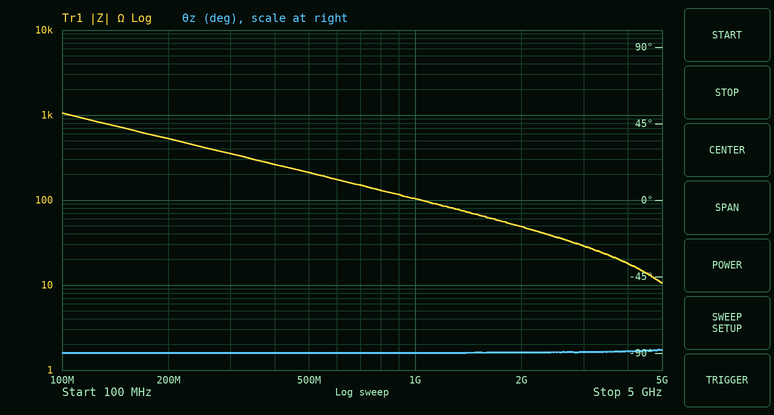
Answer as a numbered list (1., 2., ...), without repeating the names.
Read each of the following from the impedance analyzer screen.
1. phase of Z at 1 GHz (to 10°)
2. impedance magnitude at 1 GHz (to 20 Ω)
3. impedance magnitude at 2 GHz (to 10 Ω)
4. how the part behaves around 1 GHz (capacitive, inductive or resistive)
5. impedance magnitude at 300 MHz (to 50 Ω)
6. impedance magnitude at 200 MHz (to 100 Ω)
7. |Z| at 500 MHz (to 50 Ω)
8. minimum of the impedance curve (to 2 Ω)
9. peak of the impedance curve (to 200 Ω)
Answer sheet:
1. -90°
2. 100 Ω
3. 50 Ω
4. capacitive
5. 350 Ω
6. 500 Ω
7. 200 Ω
8. 10 Ω
9. 1.0 kΩ
